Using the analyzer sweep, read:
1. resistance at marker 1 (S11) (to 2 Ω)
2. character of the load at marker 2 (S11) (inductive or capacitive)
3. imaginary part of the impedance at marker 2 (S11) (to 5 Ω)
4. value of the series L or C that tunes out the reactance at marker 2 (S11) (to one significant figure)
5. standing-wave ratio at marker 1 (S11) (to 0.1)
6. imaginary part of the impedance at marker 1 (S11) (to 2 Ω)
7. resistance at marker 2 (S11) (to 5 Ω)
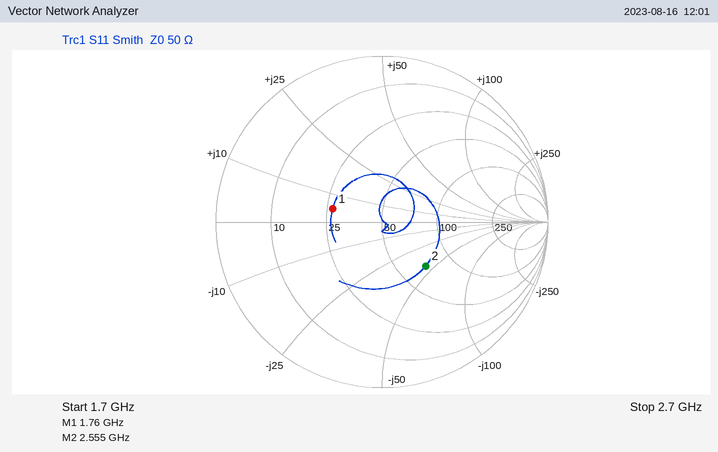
26 Ω
capacitive
-45 Ω
3 nH
1.9
+4 Ω
70 Ω
